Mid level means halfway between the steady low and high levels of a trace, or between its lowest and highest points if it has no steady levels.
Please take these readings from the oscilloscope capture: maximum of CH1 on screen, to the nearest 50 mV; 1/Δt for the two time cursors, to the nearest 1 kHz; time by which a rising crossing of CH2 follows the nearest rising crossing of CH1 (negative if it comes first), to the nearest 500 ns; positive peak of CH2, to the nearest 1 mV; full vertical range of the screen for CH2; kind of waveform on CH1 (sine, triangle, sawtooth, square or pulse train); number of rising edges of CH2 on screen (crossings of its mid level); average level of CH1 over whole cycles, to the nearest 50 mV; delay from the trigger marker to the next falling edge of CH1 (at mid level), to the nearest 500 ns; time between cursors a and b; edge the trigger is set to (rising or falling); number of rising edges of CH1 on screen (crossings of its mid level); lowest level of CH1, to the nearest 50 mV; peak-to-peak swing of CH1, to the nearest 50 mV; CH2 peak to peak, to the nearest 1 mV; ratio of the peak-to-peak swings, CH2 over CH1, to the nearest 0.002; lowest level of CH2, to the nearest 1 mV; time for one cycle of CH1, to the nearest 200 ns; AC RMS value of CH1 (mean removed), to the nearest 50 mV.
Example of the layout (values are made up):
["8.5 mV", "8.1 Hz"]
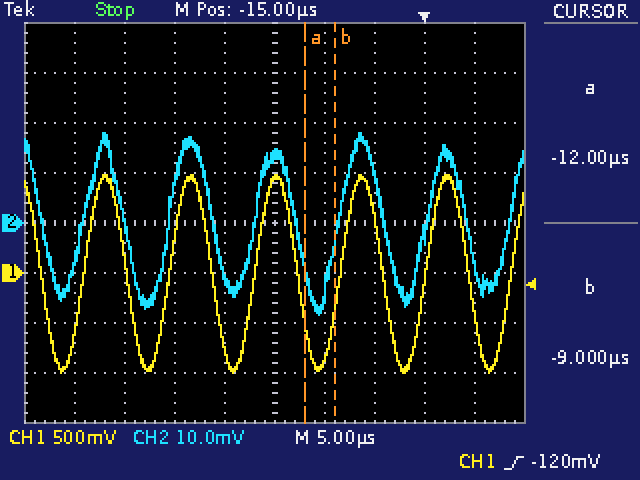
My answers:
["1.00 V", "333 kHz", "0.0 µs", "18 mV", "80 mV", "sine", "6", "0 mV", "4.5 µs", "3.0 µs", "rising", "6", "-1.00 V", "2.00 V", "36 mV", "0.018", "-18 mV", "8.6 µs", "700 mV"]
